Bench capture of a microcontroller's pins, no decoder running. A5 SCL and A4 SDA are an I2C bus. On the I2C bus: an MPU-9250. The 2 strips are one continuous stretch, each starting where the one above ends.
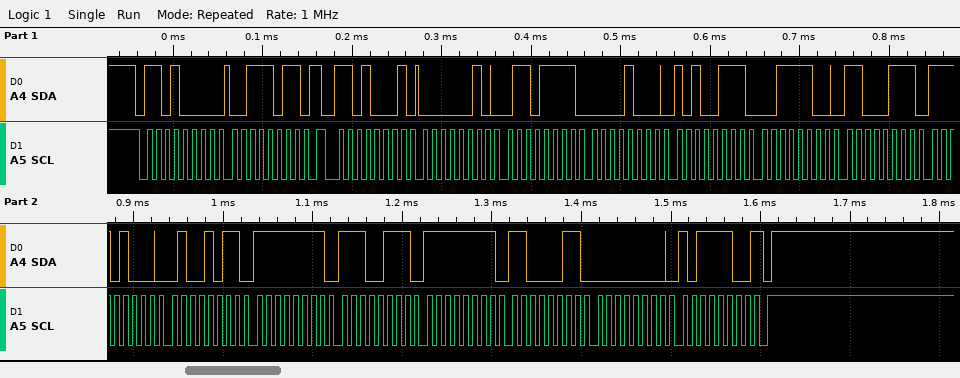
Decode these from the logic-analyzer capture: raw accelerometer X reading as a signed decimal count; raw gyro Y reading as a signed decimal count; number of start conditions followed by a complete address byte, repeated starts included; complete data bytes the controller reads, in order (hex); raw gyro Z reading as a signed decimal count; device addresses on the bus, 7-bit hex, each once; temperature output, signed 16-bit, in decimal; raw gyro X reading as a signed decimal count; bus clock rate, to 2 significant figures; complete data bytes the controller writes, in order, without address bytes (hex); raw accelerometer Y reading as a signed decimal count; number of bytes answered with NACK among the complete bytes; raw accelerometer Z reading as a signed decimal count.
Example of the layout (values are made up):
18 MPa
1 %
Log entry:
623
-61
2
02 6F 08 A7 3C C7 E8 4B FF E7 FF C3 00 BC
188
0x68
-6069
-25
100 kHz
3B
2215
1
15559
